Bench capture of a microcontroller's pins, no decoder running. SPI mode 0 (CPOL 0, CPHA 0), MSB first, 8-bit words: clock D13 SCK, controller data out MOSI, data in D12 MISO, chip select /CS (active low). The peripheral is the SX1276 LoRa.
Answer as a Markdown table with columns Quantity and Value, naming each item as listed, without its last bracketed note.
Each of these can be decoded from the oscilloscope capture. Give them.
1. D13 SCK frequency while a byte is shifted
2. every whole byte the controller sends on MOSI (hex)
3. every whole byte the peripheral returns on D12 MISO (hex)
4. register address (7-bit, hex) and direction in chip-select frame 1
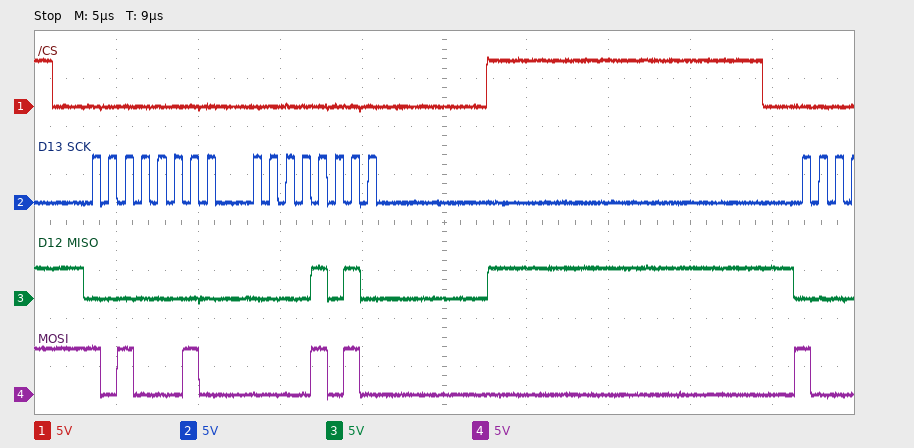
| Quantity | Value |
|---|---|
| D13 SCK frequency while a byte is shifted | 1 MHz |
| every whole byte the controller sends on MOSI | A2 0A |
| every whole byte the peripheral returns on D12 MISO | 00 0A |
| register address (7-bit, hex) and direction in chip-select frame 1 | 0x22 write |
